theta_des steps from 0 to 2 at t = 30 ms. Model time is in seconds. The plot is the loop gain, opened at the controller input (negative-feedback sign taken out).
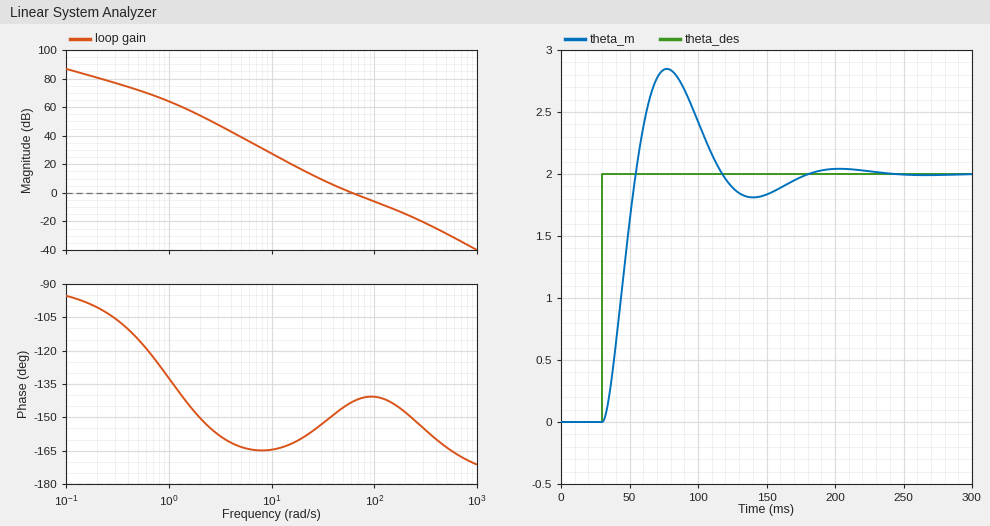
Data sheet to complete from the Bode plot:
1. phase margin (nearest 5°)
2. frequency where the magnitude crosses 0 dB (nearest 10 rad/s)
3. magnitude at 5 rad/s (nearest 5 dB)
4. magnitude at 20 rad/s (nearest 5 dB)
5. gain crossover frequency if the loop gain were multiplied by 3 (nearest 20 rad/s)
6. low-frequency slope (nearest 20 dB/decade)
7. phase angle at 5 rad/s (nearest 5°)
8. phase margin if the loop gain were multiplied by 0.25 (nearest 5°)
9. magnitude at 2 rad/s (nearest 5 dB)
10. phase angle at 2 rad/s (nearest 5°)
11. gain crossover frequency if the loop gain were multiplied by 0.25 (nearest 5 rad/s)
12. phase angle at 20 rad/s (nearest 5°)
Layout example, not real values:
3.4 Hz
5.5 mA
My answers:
35°
60 rad/s
40 dB
15 dB
140 rad/s
-20 dB/decade
-165°
25°
55 dB
-150°
25 rad/s
-160°
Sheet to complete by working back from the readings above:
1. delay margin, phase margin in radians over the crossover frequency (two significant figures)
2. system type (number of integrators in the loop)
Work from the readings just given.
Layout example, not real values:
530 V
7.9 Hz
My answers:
0.010 s
1
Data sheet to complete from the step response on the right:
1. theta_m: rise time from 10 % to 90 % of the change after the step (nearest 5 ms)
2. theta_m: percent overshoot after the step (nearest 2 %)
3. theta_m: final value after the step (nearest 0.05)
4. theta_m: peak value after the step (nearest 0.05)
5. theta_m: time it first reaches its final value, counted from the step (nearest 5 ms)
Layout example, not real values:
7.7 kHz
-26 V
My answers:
15 ms
42 %
2.00
2.85
25 ms
